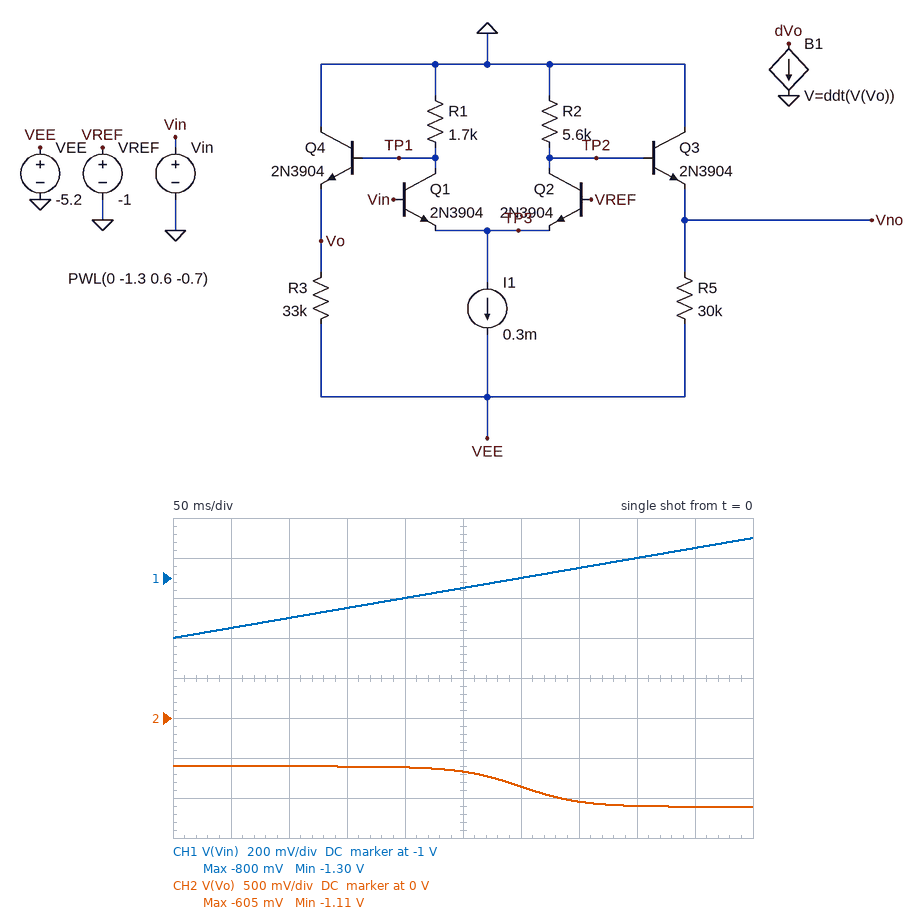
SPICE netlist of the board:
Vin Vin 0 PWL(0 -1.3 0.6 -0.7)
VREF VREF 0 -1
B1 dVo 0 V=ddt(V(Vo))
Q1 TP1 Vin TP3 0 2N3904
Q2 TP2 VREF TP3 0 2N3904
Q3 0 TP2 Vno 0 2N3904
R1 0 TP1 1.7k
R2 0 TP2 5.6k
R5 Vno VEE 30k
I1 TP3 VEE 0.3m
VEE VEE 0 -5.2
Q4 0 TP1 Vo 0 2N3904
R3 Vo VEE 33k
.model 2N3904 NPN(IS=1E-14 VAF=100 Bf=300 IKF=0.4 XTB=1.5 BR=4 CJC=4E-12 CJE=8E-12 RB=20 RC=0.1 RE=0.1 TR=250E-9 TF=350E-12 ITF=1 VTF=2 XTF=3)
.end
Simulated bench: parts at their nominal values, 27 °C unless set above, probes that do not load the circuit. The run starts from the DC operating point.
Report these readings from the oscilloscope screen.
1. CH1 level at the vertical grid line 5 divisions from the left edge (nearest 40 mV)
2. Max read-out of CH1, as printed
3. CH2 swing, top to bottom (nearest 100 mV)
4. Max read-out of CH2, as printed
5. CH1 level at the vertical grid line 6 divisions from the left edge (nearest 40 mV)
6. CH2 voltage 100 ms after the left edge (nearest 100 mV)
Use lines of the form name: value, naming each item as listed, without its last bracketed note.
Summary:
CH1 level at the vertical grid line 5 divisions from the left edge: -1.04 V
Max read-out of CH1, as printed: -800 mV
CH2 swing, top to bottom: 500 mV
Max read-out of CH2, as printed: -605 mV
CH1 level at the vertical grid line 6 divisions from the left edge: -1.00 V
CH2 voltage 100 ms after the left edge: -600 mV
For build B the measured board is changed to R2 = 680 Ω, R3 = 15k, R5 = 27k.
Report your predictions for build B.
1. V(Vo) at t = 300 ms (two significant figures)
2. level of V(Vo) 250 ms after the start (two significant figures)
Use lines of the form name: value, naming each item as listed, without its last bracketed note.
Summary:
V(Vo) at t = 300 ms: -880 mV
level of V(Vo) 250 ms after the start: -690 mV
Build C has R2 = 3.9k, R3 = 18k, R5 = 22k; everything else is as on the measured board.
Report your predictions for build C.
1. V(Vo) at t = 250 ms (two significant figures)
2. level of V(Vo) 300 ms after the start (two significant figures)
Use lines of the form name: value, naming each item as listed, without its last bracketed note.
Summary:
V(Vo) at t = 250 ms: -690 mV
level of V(Vo) 300 ms after the start: -870 mV
